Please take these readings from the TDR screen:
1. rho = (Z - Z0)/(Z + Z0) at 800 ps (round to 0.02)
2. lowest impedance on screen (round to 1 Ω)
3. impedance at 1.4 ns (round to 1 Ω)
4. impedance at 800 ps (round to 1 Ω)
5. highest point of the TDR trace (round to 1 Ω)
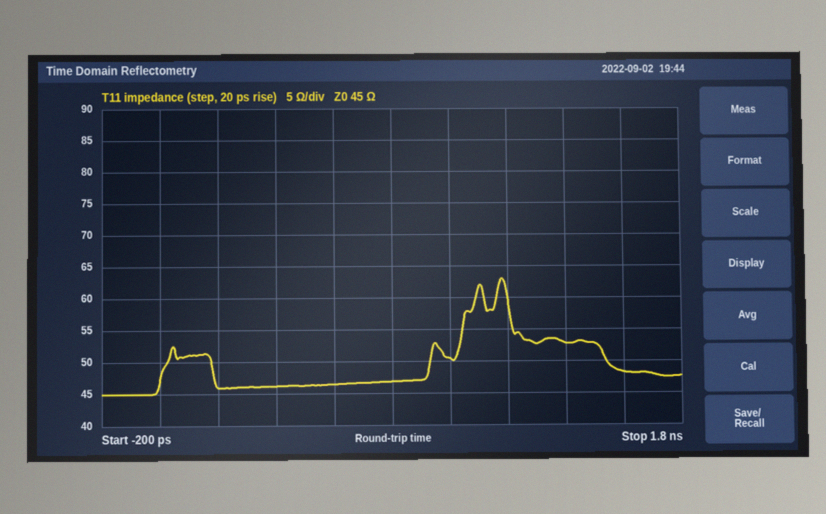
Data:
+0.02
45 Ω
53 Ω
47 Ω
63 Ω
